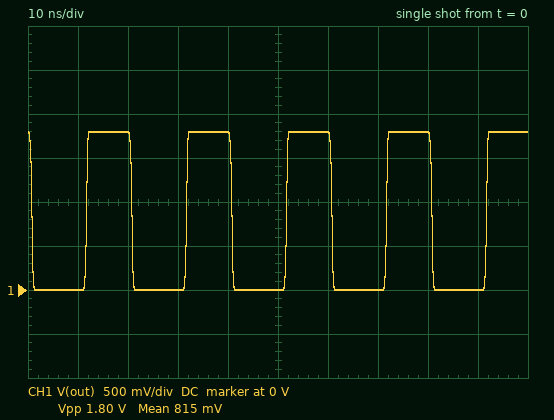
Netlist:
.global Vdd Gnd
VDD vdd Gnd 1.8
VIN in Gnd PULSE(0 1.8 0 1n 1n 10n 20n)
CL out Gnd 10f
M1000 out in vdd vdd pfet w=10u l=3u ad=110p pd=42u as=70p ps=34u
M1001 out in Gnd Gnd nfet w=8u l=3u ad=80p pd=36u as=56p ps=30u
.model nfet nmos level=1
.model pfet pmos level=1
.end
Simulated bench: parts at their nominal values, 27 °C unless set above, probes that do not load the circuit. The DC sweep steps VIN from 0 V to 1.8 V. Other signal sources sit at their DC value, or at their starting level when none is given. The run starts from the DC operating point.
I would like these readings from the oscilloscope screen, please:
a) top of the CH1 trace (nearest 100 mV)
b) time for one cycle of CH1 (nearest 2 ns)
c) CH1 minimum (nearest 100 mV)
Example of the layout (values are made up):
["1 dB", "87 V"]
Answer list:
["1.8 V", "20 ns", "0 V"]
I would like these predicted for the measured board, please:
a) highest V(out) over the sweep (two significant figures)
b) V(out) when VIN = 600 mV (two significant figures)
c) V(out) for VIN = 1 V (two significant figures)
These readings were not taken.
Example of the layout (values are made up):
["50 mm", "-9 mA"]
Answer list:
["1.8 V", "1.7 V", "550 mV"]
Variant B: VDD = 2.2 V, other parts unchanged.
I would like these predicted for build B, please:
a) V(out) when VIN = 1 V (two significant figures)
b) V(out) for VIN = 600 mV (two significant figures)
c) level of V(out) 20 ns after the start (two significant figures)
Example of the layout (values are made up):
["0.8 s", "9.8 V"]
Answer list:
["1.8 V", "2.1 V", "2.2 V"]
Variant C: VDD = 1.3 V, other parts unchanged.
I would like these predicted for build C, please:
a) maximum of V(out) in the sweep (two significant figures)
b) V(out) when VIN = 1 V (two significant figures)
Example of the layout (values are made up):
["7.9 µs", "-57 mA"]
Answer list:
["1.3 V", "58 mV"]
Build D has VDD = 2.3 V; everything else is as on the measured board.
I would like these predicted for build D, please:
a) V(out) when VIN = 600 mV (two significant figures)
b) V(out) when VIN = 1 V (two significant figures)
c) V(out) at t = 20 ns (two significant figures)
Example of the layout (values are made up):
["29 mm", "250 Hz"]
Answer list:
["2.2 V", "1.9 V", "2.3 V"]
